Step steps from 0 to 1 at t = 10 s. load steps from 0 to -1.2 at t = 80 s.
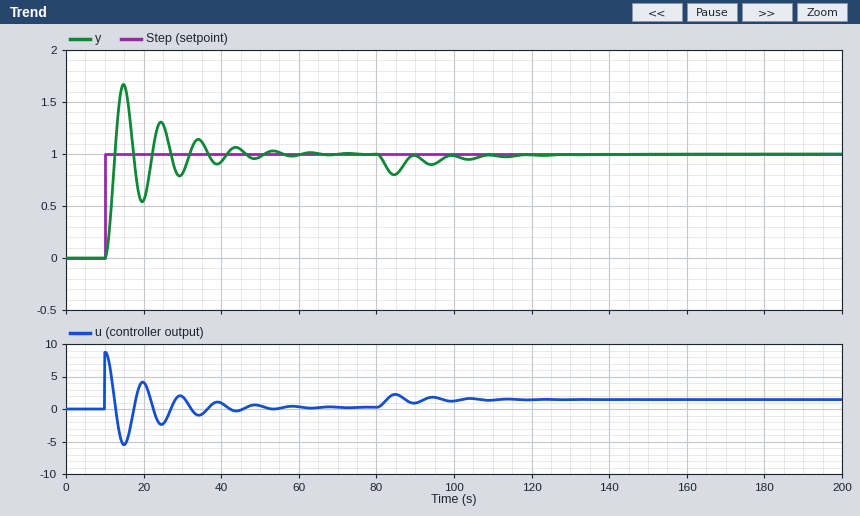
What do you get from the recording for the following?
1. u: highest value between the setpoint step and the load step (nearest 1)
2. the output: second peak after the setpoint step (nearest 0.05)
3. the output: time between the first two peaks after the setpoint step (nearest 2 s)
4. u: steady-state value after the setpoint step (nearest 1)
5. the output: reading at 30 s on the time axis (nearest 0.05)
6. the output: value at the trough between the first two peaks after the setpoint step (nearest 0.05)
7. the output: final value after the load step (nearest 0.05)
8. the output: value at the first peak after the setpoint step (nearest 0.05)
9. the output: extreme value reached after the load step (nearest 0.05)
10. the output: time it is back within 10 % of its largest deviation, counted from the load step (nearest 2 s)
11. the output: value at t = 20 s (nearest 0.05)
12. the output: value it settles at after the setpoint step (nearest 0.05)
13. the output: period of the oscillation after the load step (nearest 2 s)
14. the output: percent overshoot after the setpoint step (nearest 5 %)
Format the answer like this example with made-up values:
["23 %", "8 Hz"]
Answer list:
["9", "1.30", "10 s", "0", "0.80", "0.55", "1.00", "1.65", "0.80", "36 s", "0.55", "1.00", "10 s", "65 %"]
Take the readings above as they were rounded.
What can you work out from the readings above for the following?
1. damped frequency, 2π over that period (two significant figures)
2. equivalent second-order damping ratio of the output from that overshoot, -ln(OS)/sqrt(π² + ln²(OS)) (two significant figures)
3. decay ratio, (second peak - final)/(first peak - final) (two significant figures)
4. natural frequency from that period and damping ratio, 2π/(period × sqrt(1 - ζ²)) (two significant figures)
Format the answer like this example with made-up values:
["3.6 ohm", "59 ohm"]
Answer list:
["0.63 rad/s", "0.14", "0.46", "0.63 rad/s"]
